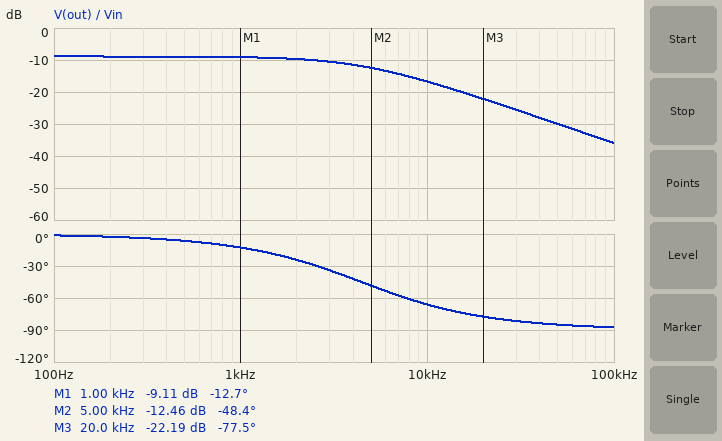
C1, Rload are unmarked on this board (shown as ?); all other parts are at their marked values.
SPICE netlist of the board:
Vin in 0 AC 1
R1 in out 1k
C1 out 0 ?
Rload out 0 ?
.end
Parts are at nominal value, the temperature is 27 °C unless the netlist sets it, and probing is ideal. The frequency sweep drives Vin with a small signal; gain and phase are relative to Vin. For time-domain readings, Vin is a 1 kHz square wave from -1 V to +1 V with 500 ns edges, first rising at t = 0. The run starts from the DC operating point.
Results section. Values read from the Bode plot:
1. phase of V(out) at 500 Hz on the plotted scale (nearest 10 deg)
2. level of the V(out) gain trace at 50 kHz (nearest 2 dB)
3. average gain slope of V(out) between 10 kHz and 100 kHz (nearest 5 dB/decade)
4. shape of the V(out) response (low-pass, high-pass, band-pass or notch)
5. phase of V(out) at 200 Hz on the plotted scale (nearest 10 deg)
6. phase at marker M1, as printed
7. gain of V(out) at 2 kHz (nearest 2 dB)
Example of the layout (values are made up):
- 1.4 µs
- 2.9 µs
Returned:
- -10 deg
- -30 dB
- -20 dB/decade
- low-pass
- 0 deg
- -12.7 deg
- -10 dB
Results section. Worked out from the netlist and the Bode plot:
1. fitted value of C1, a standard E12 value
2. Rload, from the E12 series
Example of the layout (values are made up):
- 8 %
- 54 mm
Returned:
- 100 nF
- 560 Ω
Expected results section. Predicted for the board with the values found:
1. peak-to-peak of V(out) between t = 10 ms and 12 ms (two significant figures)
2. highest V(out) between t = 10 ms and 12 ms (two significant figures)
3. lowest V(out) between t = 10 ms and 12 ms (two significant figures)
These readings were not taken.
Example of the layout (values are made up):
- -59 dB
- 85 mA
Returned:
- 720 mV
- 360 mV
- -360 mV
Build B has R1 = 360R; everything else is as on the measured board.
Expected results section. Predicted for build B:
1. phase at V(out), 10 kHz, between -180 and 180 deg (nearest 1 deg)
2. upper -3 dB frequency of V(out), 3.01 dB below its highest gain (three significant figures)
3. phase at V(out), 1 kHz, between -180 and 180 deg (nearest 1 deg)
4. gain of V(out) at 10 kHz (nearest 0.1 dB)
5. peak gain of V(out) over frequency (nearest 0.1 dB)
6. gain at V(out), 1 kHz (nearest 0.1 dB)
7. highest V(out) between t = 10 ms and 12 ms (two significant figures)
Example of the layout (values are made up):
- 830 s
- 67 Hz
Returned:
- -54 deg
- 7.26 kHz
- -8 deg
- -8.9 dB
- -4.3 dB
- -4.4 dB
- 610 mV
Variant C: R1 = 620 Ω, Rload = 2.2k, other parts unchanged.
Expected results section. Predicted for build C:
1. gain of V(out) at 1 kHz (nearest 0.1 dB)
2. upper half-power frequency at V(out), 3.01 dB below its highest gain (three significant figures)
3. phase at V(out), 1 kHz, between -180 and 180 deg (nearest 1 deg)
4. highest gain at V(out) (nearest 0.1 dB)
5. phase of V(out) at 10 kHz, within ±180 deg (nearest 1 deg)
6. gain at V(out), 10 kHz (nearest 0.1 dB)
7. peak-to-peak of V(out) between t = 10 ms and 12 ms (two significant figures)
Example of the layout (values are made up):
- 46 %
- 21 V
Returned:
- -2.5 dB
- 3.29 kHz
- -17 deg
- -2.2 dB
- -72 deg
- -12.3 dB
- 1.6 V
